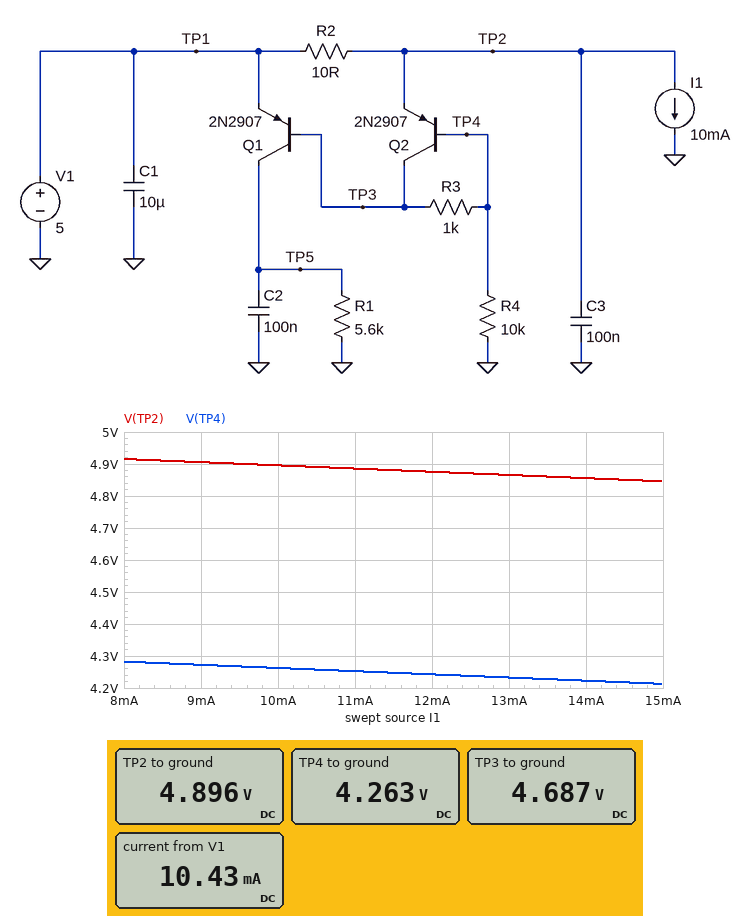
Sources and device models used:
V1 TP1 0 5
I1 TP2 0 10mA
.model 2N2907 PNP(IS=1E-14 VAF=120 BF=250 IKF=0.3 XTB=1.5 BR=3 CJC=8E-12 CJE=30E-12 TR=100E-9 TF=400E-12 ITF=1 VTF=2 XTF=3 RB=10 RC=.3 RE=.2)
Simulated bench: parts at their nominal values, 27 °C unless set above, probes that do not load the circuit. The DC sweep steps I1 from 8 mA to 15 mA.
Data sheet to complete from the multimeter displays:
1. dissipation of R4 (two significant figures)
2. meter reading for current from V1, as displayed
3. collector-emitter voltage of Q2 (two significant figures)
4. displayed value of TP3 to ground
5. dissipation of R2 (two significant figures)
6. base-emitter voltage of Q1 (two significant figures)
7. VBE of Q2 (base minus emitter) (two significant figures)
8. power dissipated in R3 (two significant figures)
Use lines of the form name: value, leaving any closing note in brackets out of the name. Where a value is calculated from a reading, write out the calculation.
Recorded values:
dissipation of R4: (4.263 V)^2 / 10 kΩ = 1.8 mW
meter reading for current from V1, as displayed: 10.43 mA
collector-emitter voltage of Q2: 4.687 V - 4.896 V = -210 mV
displayed value of TP3 to ground: 4.687 V
dissipation of R2: (5 V - 4.896 V)^2 / 10 Ω = 1.1 mW
base-emitter voltage of Q1: 4.687 V - 5 V = -310 mV
VBE of Q2 (base minus emitter): 4.263 V - 4.896 V = -630 mV
power dissipated in R3: (4.687 V - 4.263 V)^2 / 1 kΩ = 180 µW
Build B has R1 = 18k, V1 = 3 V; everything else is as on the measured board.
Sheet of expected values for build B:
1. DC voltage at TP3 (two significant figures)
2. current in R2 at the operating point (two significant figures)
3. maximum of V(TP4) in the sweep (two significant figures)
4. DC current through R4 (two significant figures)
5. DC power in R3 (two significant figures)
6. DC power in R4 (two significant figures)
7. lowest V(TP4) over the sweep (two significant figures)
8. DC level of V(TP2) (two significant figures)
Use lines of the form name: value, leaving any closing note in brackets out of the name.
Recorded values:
DC voltage at TP3: 2.5 V
current in R2 at the operating point: 10 mA
maximum of V(TP4) in the sweep: 2.3 V
DC current through R4: 230 µA
DC power in R3: 52 µW
DC power in R4: 520 µW
lowest V(TP4) over the sweep: 2.2 V
DC level of V(TP2): 2.9 V
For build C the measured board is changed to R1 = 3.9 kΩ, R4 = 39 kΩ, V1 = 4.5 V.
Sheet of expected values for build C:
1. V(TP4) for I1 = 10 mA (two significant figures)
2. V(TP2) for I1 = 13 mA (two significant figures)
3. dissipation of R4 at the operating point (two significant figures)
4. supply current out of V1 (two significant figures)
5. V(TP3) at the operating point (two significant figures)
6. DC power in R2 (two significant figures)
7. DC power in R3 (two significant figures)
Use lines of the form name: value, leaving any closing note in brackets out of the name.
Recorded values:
V(TP4) for I1 = 10 mA: 3.8 V
V(TP2) for I1 = 13 mA: 4.4 V
dissipation of R4 at the operating point: 370 µW
supply current out of V1: 10 mA
V(TP3) at the operating point: 3.9 V
DC power in R2: 1.0 mW
DC power in R3: 9.4 µW
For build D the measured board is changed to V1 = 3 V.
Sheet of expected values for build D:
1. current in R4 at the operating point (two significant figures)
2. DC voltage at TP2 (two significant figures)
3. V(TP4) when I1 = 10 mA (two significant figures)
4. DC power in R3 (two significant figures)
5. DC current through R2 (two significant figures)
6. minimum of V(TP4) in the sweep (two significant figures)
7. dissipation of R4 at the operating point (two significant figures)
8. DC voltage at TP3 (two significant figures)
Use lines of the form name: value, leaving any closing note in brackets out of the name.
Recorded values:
current in R4 at the operating point: 230 µA
DC voltage at TP2: 2.9 V
V(TP4) when I1 = 10 mA: 2.3 V
DC power in R3: 52 µW
DC current through R2: 10 mA
minimum of V(TP4) in the sweep: 2.2 V
dissipation of R4 at the operating point: 520 µW
DC voltage at TP3: 2.5 V
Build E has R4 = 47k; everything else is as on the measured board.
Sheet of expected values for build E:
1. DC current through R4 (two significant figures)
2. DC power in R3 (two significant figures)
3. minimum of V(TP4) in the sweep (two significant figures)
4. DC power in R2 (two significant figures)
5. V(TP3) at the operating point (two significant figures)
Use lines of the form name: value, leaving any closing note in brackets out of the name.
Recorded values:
DC current through R4: 92 µA
DC power in R3: 8.3 µW
minimum of V(TP4) in the sweep: 4.3 V
DC power in R2: 1.0 mW
V(TP3) at the operating point: 4.4 V
